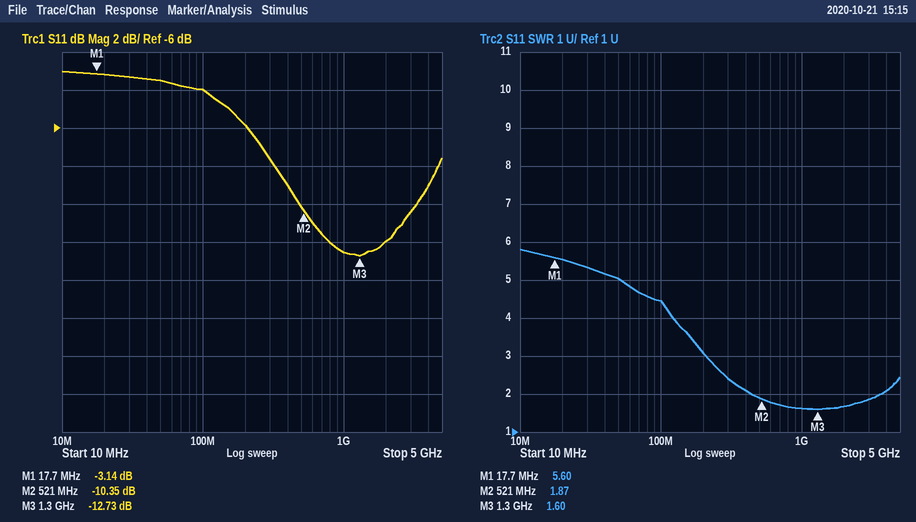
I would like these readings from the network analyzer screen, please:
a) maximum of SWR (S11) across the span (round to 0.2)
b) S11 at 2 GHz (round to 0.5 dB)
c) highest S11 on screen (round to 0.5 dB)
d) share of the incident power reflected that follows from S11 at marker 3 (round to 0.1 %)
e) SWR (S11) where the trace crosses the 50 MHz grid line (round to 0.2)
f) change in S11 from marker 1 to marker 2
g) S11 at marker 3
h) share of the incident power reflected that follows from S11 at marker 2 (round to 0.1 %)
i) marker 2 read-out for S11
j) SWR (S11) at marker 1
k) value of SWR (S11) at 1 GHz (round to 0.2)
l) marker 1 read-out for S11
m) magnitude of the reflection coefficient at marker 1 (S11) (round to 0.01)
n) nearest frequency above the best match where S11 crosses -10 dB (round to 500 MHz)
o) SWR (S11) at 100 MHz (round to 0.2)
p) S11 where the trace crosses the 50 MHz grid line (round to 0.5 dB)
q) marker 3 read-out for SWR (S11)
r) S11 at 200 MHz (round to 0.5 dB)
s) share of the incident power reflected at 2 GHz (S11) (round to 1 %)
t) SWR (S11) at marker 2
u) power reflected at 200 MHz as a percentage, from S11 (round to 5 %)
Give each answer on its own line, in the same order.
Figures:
5.8
-12.0 dB
-3.0 dB
5.3 %
5.0
-7.21 dB
-12.73 dB
9.2 %
-10.35 dB
5.60
1.6
-3.14 dB
0.70
3.5 GHz
4.4
-3.5 dB
1.60
-6.0 dB
6 %
1.87
25 %
